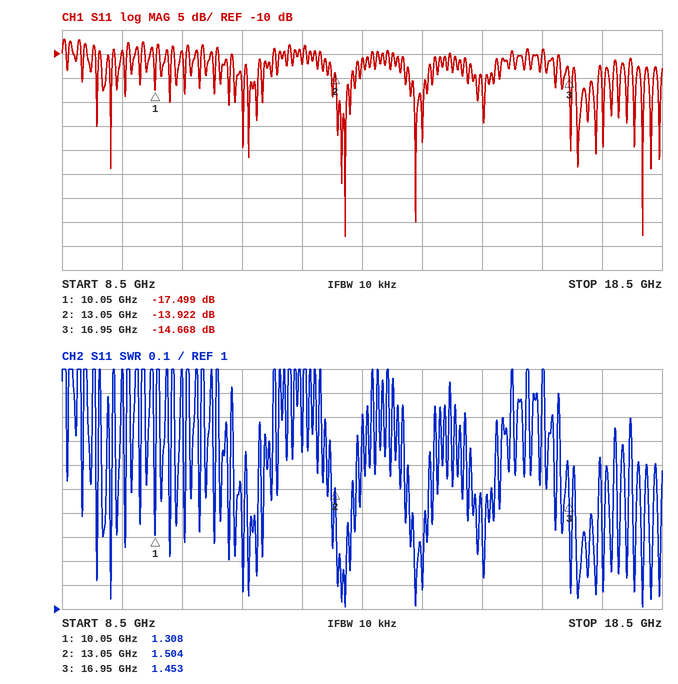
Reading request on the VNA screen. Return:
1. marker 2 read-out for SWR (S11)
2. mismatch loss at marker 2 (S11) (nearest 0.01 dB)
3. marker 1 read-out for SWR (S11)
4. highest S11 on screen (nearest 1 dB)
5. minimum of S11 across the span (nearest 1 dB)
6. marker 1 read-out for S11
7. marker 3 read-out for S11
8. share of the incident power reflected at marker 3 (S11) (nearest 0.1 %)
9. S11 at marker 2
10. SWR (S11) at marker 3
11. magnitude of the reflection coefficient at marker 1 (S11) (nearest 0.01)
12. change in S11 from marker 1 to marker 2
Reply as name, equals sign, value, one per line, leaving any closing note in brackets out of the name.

marker 2 read-out for SWR = 1.504
mismatch loss at marker 2 (S11) = 0.18 dB
marker 1 read-out for SWR = 1.308
highest S11 on screen = -7 dB
minimum of S11 across the span = -48 dB
marker 1 read-out for S11 = -17.499 dB
marker 3 read-out for S11 = -14.668 dB
share of the incident power reflected at marker 3 (S11) = 3.4 %
S11 at marker 2 = -13.922 dB
SWR (S11) at marker 3 = 1.453
magnitude of the reflection coefficient at marker 1 (S11) = 0.13
change in S11 from marker 1 to marker 2 = 3.577 dB
